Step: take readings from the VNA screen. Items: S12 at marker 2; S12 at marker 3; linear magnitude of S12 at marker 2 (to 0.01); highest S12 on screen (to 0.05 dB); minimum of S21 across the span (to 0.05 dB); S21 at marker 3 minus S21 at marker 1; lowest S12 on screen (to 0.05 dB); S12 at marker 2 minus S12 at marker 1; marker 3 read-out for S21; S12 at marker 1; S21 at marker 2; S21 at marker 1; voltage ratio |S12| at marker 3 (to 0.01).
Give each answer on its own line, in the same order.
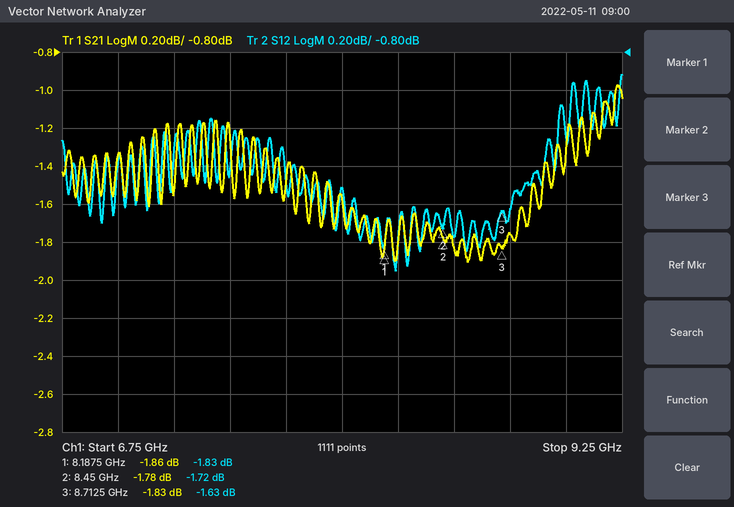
-1.72 dB
-1.63 dB
0.82
-0.90 dB
-1.90 dB
0.03 dB
-1.95 dB
0.11 dB
-1.83 dB
-1.83 dB
-1.78 dB
-1.86 dB
0.83
